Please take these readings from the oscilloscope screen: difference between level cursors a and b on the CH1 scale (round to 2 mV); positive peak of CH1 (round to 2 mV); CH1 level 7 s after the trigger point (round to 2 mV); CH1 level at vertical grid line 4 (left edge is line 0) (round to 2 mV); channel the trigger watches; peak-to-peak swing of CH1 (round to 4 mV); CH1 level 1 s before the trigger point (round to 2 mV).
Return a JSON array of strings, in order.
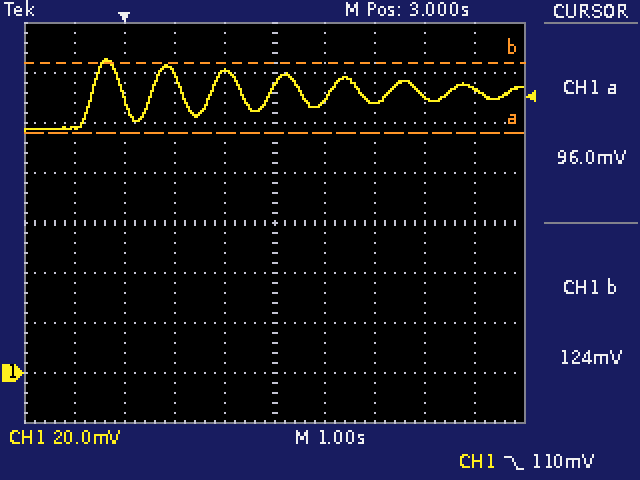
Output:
["28 mV", "126 mV", "114 mV", "120 mV", "CH1", "28 mV", "98 mV"]
